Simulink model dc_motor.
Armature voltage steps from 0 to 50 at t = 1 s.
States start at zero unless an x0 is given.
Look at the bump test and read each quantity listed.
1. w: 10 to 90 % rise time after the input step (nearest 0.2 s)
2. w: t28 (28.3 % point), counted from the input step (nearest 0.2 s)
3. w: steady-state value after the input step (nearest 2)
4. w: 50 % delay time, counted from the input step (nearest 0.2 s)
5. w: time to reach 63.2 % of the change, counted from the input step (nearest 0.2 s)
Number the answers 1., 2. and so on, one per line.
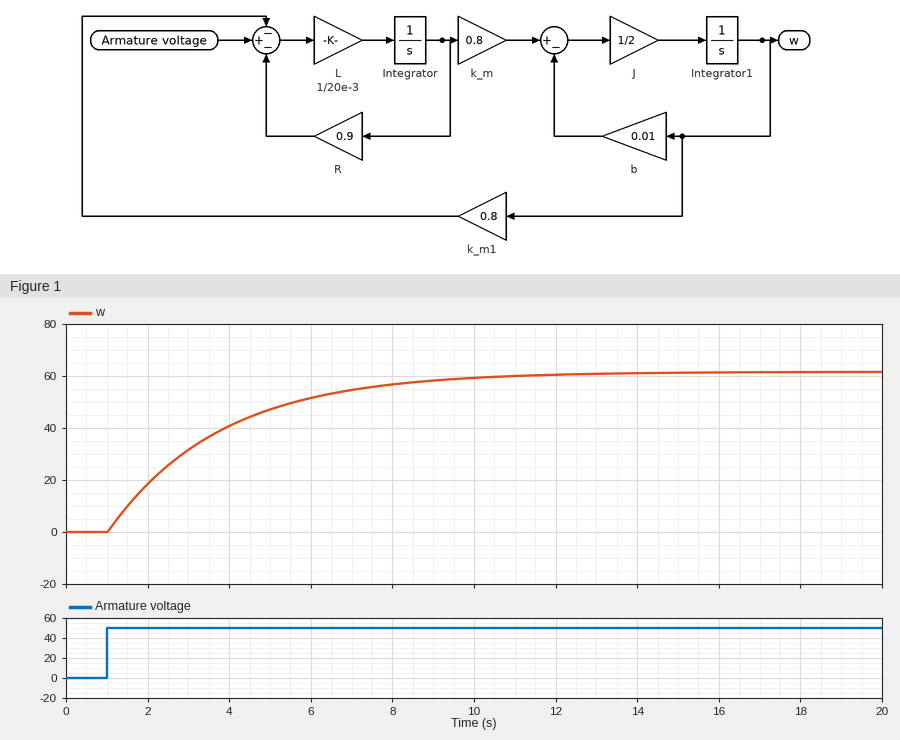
1. 6.0 s
2. 1.0 s
3. 62
4. 2.0 s
5. 2.8 s
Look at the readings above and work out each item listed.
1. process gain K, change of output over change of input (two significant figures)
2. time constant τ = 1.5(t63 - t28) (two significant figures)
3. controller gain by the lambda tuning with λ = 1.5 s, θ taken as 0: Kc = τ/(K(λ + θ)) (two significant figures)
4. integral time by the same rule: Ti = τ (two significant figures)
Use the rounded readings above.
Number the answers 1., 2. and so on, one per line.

1. 1.2
2. 2.7 s
3. 1.5
4. 2.7 s
